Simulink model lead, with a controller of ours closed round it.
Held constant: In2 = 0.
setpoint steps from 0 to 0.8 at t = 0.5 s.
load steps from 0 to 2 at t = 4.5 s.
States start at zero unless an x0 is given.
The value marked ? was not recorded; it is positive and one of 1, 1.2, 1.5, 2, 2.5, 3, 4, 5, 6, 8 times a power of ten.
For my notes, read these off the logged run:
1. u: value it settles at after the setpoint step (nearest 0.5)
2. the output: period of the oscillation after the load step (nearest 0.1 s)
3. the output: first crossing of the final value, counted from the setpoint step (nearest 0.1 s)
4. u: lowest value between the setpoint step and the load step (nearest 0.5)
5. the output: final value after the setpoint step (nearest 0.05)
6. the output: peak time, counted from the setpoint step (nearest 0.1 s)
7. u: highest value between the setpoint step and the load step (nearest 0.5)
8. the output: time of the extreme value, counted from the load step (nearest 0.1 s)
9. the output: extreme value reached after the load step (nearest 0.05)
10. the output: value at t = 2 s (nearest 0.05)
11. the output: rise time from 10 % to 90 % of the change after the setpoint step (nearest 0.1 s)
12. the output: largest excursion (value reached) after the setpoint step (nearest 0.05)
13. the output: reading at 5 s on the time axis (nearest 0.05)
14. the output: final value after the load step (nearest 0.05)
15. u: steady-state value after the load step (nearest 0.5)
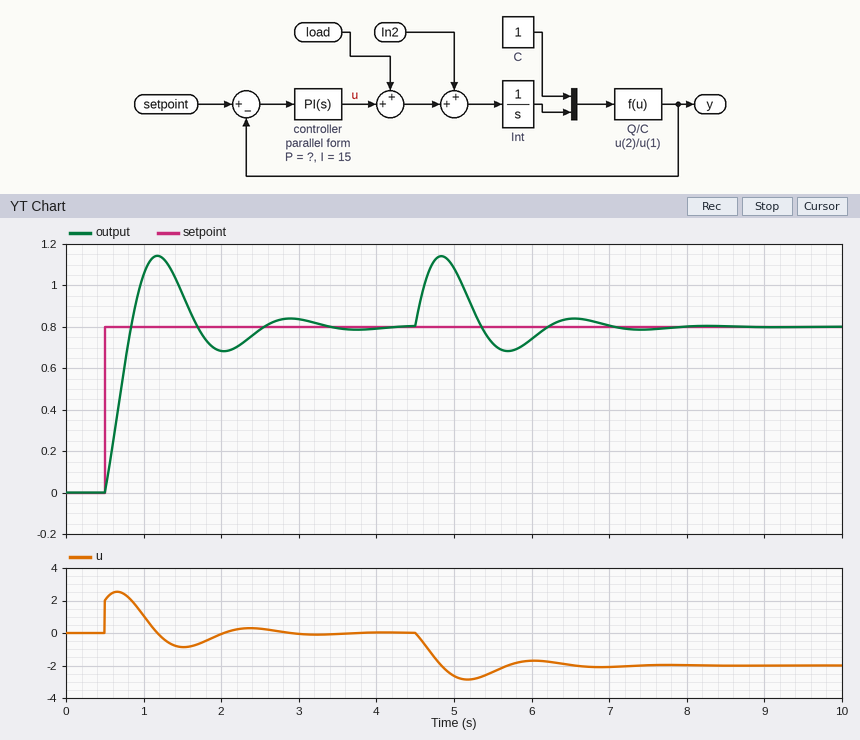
0.0
1.7 s
0.3 s
-1.0
0.80
0.7 s
2.5
0.3 s
1.15
0.70
0.3 s
1.15
1.10
0.80
-2.0
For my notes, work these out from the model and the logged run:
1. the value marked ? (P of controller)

2.5
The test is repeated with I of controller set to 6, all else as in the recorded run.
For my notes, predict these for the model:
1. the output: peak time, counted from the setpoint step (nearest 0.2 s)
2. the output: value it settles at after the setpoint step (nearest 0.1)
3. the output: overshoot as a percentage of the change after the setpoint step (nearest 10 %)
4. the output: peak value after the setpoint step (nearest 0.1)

1.0 s
0.8
30 %
1.0
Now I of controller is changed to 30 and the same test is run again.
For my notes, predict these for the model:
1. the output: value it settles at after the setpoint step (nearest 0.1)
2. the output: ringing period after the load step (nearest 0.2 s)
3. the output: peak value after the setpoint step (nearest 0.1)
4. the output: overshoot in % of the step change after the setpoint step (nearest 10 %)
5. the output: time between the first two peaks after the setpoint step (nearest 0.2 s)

0.8
1.2 s
1.2
50 %
1.2 s
